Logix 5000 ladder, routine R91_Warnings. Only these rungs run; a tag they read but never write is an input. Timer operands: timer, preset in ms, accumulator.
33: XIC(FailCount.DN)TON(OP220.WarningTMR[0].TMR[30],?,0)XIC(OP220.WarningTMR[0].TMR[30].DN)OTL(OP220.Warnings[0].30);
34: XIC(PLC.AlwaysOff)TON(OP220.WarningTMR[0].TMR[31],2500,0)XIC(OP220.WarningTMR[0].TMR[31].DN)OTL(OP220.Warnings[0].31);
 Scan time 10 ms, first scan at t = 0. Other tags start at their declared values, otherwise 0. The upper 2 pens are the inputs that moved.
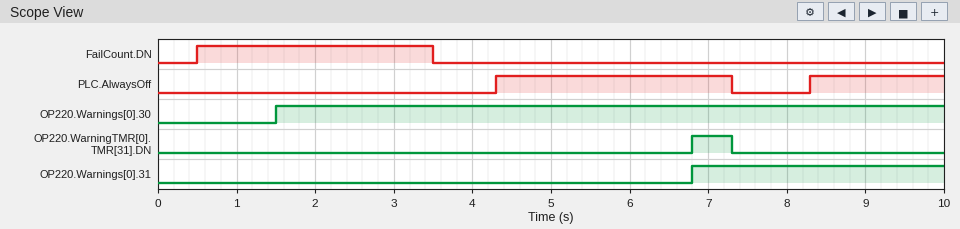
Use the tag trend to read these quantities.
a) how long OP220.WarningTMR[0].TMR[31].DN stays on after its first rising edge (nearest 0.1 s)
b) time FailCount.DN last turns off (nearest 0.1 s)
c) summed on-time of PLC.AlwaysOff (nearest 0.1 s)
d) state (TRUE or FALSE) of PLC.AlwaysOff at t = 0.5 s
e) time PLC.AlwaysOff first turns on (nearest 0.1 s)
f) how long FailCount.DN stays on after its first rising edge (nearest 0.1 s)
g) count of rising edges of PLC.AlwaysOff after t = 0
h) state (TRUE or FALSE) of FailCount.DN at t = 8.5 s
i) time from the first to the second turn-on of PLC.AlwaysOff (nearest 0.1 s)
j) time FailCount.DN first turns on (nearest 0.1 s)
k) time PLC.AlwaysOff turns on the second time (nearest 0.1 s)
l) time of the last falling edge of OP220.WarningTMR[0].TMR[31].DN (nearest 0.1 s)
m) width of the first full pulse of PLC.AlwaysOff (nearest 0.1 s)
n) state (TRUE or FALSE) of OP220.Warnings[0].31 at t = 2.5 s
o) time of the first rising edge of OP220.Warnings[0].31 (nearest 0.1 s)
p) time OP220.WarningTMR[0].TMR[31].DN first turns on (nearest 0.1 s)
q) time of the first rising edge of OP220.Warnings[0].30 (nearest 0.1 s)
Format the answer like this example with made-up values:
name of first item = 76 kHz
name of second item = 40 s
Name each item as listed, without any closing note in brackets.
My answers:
how long OP220.WarningTMR[0].TMR[31].DN stays on after its first rising edge = 0.5 s
time FailCount.DN last turns off = 3.5 s
summed on-time of PLC.AlwaysOff = 4.7 s
state (TRUE or FALSE) of PLC.AlwaysOff at t = 0.5 s = FALSE
time PLC.AlwaysOff first turns on = 4.3 s
how long FailCount.DN stays on after its first rising edge = 3.0 s
count of rising edges of PLC.AlwaysOff after t = 0 = 2
state (TRUE or FALSE) of FailCount.DN at t = 8.5 s = FALSE
time from the first to the second turn-on of PLC.AlwaysOff = 4.0 s
time FailCount.DN first turns on = 0.5 s
time PLC.AlwaysOff turns on the second time = 8.3 s
time of the last falling edge of OP220.WarningTMR[0].TMR[31].DN = 7.3 s
width of the first full pulse of PLC.AlwaysOff = 3.0 s
state (TRUE or FALSE) of OP220.Warnings[0].31 at t = 2.5 s = FALSE
time of the first rising edge of OP220.Warnings[0].31 = 6.8 s
time OP220.WarningTMR[0].TMR[31].DN first turns on = 6.8 s
time of the first rising edge of OP220.Warnings[0].30 = 1.5 s
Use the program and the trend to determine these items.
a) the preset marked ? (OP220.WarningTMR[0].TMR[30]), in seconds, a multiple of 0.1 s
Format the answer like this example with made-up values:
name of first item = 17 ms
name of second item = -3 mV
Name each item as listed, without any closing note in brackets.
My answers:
the preset marked ? (OP220.WarningTMR[0].TMR[30]), in seconds, a multiple of 0.1 s = 1.0 s
